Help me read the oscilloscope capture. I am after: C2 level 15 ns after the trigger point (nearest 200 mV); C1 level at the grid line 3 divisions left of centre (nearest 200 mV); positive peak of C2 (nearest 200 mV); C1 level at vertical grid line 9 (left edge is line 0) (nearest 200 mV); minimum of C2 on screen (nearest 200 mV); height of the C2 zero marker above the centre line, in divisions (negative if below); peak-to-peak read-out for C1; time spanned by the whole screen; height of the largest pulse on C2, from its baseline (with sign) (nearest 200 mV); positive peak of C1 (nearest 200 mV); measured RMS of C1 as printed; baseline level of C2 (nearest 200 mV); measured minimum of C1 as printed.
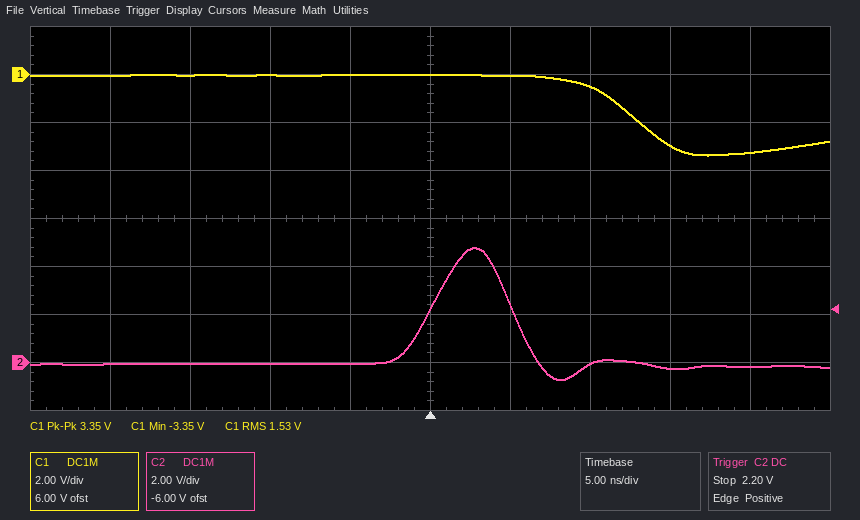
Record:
-200 mV
0.0 V
4.8 V
-3.2 V
-800 mV
-3.0 div
3.35 V
50 ns
+4.8 V
0.0 V
1.53 V
0.0 V
-3.35 V
